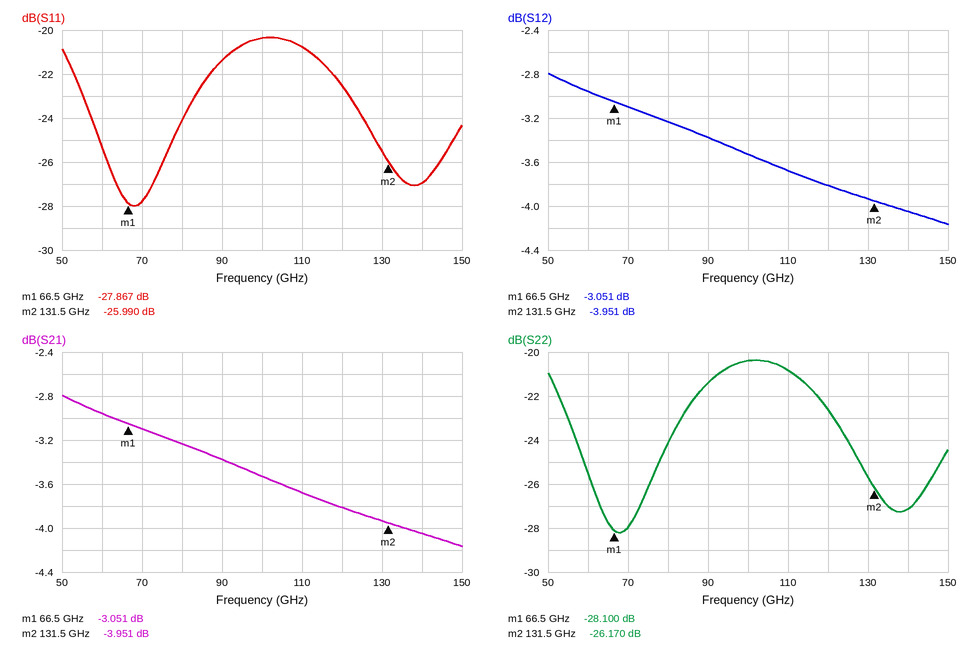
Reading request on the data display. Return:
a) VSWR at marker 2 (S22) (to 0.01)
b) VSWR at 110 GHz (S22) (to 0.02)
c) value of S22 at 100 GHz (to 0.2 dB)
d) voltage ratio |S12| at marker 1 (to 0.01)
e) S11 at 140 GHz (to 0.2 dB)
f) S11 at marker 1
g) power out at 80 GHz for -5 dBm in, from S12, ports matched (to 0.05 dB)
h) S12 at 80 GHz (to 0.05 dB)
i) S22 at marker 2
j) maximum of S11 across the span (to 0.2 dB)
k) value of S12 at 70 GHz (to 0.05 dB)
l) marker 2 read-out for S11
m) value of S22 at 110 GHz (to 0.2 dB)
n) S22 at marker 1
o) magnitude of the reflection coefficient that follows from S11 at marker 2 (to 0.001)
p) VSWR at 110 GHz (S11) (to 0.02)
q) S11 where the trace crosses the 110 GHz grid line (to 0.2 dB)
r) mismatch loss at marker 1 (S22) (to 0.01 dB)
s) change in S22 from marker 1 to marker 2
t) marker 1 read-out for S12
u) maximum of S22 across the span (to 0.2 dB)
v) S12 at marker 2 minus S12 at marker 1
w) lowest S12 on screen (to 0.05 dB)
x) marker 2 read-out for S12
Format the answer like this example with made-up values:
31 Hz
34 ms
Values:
1.10
1.20
-20.4 dB
0.70
-27.0 dB
-27.867 dB
-8.25 dBm
-3.25 dB
-26.170 dB
-20.4 dB
-3.10 dB
-25.990 dB
-20.8 dB
-28.100 dB
0.050
1.20
-20.8 dB
0.01 dB
1.930 dB
-3.051 dB
-20.4 dB
-0.900 dB
-4.15 dB
-3.951 dB
